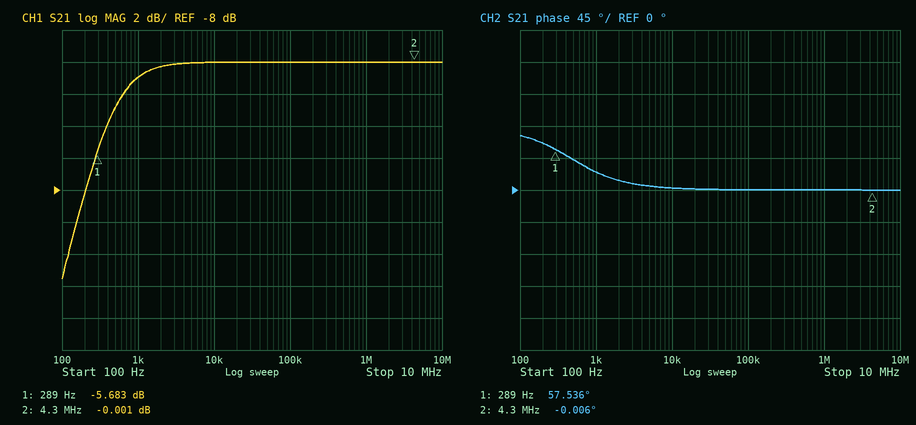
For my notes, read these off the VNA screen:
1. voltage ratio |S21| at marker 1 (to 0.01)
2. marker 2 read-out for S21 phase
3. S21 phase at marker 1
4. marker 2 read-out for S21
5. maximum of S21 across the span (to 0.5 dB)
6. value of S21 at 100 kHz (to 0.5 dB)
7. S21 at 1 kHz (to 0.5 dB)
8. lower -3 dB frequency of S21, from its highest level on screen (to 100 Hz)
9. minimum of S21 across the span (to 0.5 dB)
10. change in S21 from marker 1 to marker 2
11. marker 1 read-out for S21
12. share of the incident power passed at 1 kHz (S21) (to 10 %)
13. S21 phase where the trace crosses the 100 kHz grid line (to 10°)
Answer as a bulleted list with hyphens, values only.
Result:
- 0.52
- -0.006°
- 57.536°
- -0.001 dB
- 0.0 dB
- 0.0 dB
- -1.0 dB
- 500 Hz
- -13.5 dB
- 5.682 dB
- -5.683 dB
- 80 %
- 0°
